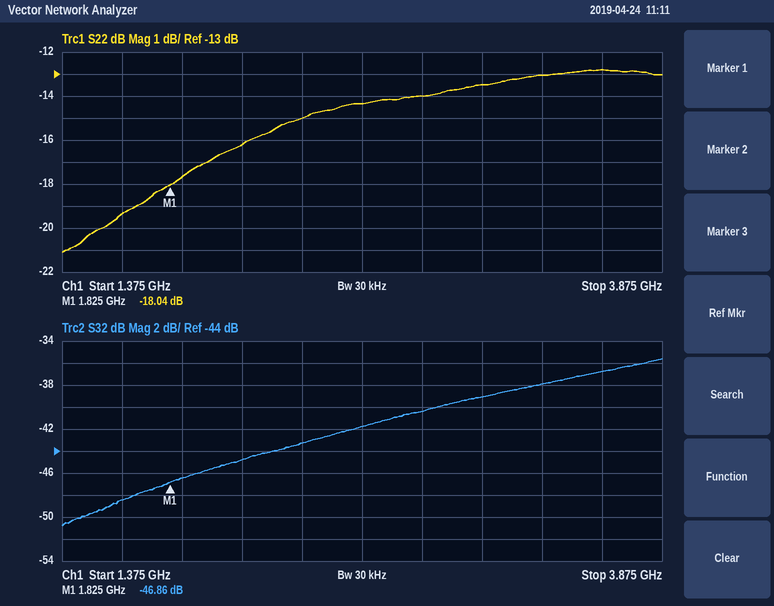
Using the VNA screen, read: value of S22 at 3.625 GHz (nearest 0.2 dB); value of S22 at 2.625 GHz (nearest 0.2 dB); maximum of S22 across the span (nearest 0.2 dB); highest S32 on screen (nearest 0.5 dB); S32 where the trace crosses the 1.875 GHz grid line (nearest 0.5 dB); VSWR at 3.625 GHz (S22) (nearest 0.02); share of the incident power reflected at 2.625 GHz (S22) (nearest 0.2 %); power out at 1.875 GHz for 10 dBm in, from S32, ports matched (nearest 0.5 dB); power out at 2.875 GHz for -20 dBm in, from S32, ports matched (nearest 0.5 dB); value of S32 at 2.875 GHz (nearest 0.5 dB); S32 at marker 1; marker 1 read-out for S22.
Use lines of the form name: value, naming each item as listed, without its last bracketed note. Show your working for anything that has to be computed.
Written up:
value of S22 at 3.625 GHz: -12.8 dB
value of S22 at 2.625 GHz: -14.4 dB
maximum of S22 across the span: -12.8 dB
highest S32 on screen: -35.5 dB
S32 where the trace crosses the 1.875 GHz grid line: -46.5 dB
VSWR at 3.625 GHz (S22): |Γ| = 10^(-12.8/20) = 0.2291; VSWR = (1 + 0.2291)/(1 − 0.2291) ≈ 1.59, so 1.60 to the nearest 0.02
share of the incident power reflected at 2.625 GHz (S22): 10^(-14.4/10) ≈ 3.6 %
power out at 1.875 GHz for 10 dBm in, from S32, ports matched: 10 dBm + (-46.5 dB) = -36.5 dBm
power out at 2.875 GHz for -20 dBm in, from S32, ports matched: -20 dBm + (-40.5 dB) = -60.5 dBm
value of S32 at 2.875 GHz: -40.5 dB
S32 at marker 1: -46.86 dB
marker 1 read-out for S22: -18.04 dB
